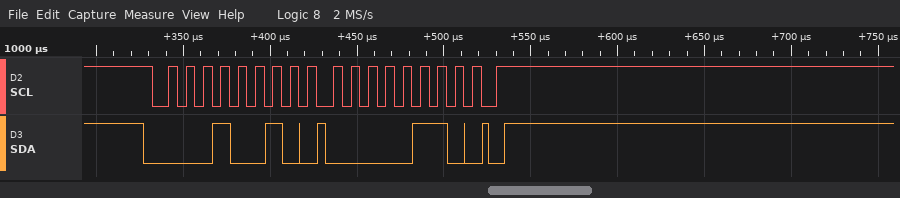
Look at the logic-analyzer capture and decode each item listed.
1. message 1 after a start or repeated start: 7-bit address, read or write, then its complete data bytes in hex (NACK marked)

0x09 write: 06
